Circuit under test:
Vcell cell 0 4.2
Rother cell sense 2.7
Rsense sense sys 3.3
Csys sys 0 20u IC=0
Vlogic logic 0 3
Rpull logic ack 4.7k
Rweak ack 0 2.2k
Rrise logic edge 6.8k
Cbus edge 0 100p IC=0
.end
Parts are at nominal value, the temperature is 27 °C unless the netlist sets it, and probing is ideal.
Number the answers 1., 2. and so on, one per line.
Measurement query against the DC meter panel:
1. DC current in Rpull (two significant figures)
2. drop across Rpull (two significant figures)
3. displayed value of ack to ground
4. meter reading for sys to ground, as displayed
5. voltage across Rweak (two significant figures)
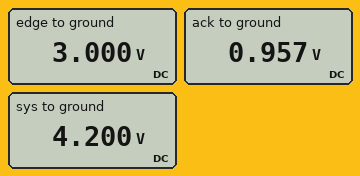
1. 430 µA
2. 2.0 V
3. 0.957 V
4. 4.200 V
5. 960 mV
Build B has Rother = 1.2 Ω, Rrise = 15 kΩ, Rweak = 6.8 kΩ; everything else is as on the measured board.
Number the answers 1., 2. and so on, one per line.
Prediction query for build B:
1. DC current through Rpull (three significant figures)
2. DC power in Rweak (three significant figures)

1. 261 µA
2. 463 µW
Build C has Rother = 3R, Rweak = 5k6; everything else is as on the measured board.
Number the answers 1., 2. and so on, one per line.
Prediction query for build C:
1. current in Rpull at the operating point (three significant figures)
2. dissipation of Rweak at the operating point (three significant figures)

1. 291 µA
2. 475 µW
